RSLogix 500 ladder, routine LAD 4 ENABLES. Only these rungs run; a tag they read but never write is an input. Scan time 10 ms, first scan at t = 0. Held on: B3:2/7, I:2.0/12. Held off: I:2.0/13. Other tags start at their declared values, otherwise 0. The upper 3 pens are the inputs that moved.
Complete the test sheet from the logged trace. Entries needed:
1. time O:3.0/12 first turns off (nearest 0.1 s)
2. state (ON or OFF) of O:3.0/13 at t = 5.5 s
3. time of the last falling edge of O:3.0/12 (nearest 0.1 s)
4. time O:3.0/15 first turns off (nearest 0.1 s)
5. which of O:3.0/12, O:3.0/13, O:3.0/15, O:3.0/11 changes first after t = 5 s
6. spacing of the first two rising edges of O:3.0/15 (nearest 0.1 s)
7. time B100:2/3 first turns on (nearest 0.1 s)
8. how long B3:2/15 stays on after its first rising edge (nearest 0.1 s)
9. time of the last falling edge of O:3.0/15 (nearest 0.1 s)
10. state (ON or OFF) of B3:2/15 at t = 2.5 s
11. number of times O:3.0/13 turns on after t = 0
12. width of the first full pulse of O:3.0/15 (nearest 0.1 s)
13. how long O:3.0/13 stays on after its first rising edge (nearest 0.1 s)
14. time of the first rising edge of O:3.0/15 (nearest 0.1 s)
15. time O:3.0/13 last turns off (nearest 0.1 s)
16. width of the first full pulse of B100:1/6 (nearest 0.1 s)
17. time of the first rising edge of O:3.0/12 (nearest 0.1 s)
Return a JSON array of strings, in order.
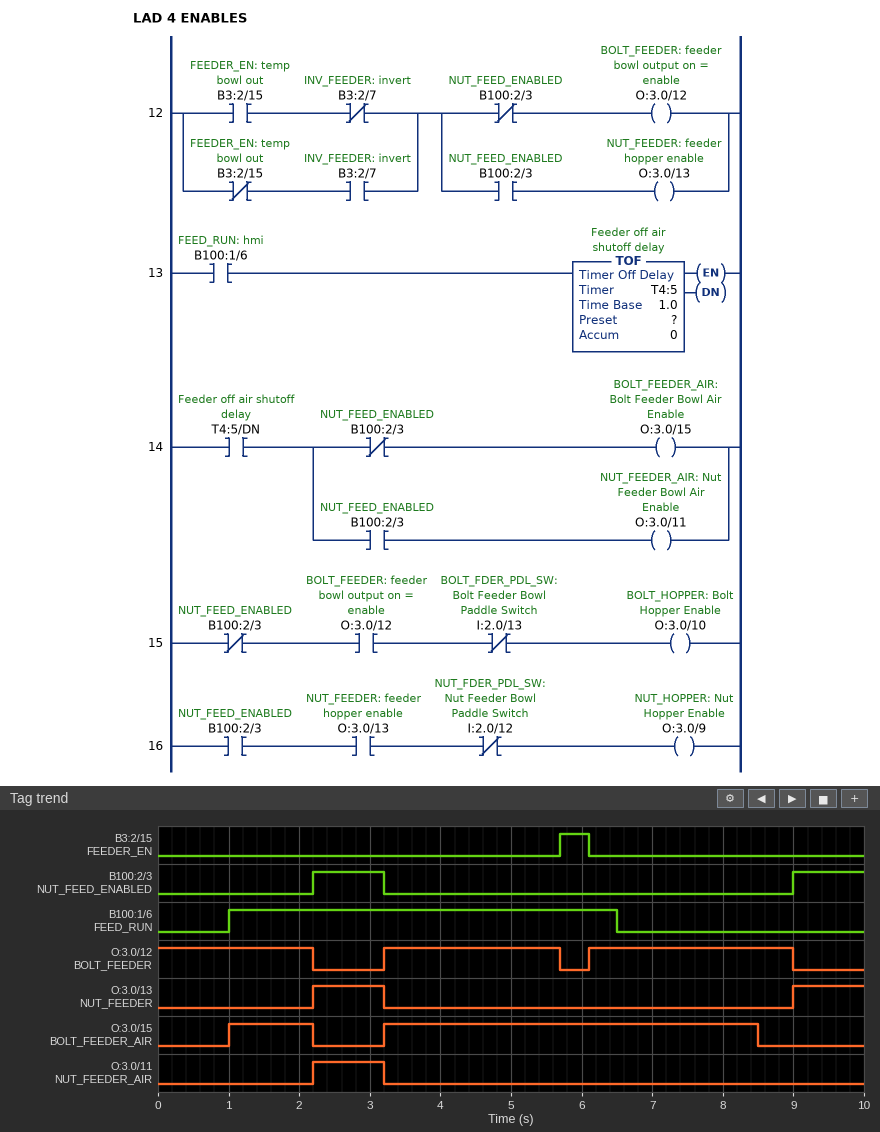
["2.2 s", "OFF", "9.0 s", "2.2 s", "O:3.0/12", "2.2 s", "2.2 s", "0.4 s", "8.5 s", "OFF", "2", "1.2 s", "1.0 s", "1.0 s", "3.2 s", "5.5 s", "3.2 s"]
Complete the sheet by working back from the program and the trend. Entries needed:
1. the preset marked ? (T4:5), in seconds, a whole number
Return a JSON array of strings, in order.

["2 s"]
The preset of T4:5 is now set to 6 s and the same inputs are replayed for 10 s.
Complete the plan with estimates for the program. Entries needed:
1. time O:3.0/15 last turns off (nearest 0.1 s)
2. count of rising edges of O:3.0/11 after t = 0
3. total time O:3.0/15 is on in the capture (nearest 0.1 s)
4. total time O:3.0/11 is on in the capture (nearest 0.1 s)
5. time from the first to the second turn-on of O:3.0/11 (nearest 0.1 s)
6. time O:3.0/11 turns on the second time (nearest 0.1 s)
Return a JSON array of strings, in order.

["9.0 s", "2", "7.0 s", "2.0 s", "6.8 s", "9.0 s"]
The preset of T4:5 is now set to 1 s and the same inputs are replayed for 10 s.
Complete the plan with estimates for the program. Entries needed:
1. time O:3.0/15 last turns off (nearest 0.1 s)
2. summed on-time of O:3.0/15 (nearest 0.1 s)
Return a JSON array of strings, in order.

["7.5 s", "5.5 s"]
